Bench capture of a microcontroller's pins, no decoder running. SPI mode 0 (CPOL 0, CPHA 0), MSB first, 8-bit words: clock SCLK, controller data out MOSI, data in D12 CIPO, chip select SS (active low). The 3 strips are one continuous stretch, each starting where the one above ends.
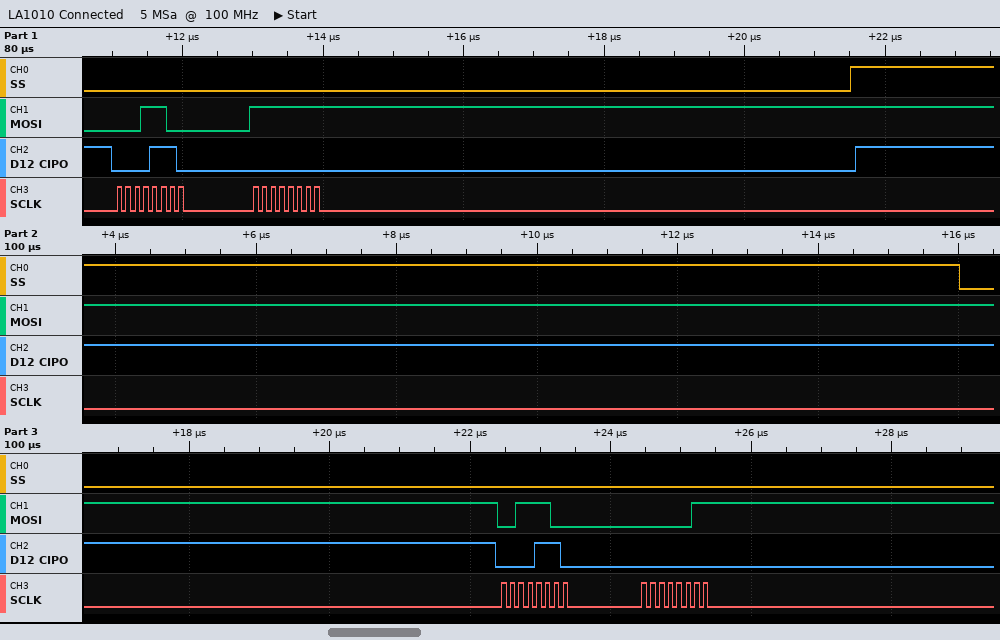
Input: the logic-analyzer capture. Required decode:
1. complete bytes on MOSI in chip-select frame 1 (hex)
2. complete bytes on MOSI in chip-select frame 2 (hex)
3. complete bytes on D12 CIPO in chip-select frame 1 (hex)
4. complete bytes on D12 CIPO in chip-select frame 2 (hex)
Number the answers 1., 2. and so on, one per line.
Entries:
1. 1C FF
2. 3C 03
3. 0E 00
4. 0E 00
